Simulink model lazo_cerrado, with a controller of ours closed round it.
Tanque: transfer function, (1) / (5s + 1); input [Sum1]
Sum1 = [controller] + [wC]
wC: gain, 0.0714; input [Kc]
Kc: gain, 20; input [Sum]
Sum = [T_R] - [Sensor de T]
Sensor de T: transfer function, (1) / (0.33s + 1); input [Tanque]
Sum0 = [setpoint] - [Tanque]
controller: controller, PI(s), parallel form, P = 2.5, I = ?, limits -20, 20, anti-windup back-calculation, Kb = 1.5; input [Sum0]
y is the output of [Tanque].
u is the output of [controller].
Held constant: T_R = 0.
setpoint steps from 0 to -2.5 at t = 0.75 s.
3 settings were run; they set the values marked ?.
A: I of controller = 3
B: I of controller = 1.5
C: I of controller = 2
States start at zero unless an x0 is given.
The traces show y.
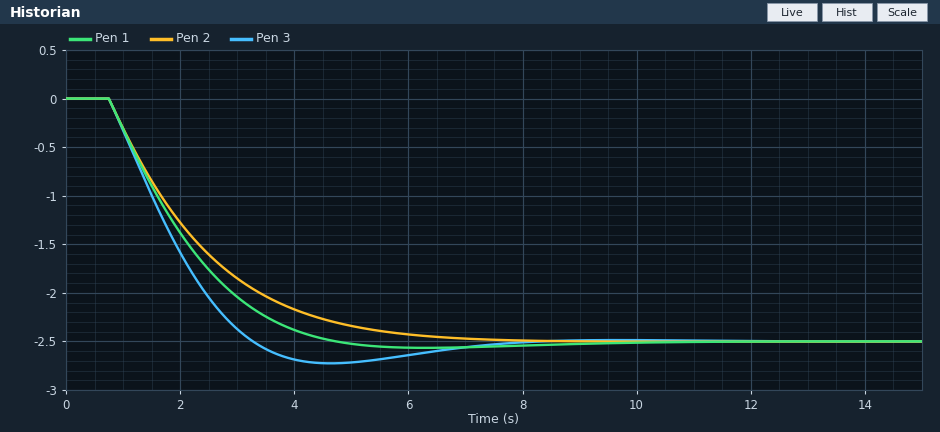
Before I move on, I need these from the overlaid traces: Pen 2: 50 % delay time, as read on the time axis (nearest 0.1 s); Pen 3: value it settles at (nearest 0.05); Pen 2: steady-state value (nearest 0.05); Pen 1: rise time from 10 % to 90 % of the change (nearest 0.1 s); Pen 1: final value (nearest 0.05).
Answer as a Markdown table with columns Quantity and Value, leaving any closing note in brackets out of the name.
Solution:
| Quantity | Value |
|---|---|
| Pen 2: 50 % delay time, as read on the time axis | 2.0 s |
| Pen 3: value it settles at | -2.50 |
| Pen 2: steady-state value | -2.50 |
| Pen 1: rise time from 10 % to 90 % of the change | 2.6 s |
| Pen 1: final value | -2.50 |
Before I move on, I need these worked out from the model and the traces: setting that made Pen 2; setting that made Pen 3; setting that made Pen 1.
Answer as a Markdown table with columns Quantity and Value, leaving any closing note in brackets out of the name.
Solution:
| Quantity | Value |
|---|---|
| setting that made Pen 2 | B |
| setting that made Pen 3 | A |
| setting that made Pen 1 | C |
